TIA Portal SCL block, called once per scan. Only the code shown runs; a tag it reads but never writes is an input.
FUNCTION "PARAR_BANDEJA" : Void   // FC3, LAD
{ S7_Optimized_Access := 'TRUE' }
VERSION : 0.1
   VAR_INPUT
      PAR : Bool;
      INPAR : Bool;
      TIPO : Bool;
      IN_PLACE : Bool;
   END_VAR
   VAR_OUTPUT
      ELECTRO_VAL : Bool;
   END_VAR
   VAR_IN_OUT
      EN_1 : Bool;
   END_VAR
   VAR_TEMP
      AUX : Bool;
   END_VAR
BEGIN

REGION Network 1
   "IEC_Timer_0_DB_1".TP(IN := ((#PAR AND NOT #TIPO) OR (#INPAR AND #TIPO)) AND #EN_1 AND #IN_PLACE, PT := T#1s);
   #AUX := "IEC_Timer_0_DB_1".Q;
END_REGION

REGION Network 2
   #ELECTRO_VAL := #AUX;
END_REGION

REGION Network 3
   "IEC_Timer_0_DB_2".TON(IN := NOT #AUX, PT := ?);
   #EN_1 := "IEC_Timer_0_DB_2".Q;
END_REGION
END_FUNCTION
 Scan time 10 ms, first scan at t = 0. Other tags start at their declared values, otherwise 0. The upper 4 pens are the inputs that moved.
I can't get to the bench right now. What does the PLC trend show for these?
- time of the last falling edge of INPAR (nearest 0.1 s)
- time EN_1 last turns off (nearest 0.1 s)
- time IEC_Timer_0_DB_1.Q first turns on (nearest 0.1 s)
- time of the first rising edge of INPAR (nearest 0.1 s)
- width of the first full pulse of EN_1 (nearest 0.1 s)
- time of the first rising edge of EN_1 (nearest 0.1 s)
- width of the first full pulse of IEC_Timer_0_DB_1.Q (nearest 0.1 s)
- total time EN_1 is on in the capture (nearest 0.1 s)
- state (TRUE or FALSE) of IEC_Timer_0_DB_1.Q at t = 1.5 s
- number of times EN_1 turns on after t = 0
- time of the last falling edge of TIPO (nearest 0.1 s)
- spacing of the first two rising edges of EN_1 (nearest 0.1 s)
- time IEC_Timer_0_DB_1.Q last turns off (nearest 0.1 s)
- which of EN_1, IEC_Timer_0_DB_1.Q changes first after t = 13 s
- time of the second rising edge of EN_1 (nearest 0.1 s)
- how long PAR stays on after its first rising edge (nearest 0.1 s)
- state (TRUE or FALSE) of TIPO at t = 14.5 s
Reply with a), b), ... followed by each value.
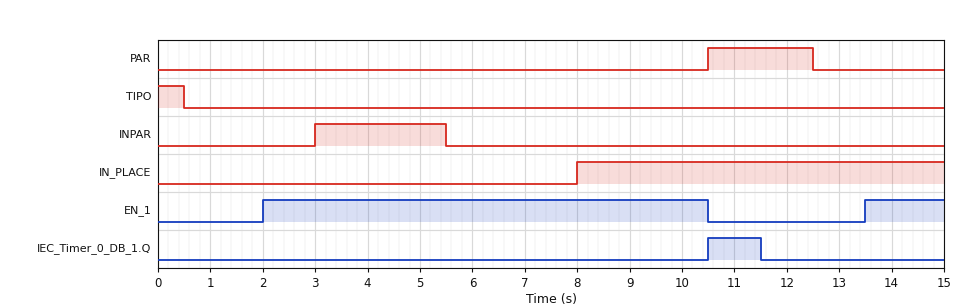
a) 5.5 s
b) 10.5 s
c) 10.5 s
d) 3.0 s
e) 8.5 s
f) 2.0 s
g) 1.0 s
h) 10.0 s
i) FALSE
j) 2
k) 0.5 s
l) 11.5 s
m) 11.5 s
n) EN_1
o) 13.5 s
p) 2.0 s
q) FALSE
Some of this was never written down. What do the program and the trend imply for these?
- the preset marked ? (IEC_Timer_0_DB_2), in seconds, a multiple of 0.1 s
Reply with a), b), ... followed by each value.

a) 2.0 s
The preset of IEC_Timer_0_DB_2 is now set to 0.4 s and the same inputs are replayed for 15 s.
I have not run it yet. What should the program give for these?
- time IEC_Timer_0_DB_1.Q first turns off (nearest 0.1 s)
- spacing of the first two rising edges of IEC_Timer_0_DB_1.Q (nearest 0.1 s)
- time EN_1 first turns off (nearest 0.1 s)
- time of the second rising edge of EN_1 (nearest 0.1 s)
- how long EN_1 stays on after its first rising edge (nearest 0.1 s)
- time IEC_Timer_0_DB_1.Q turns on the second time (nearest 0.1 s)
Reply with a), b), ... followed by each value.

a) 11.5 s
b) 1.4 s
c) 10.5 s
d) 11.9 s
e) 10.1 s
f) 11.9 s
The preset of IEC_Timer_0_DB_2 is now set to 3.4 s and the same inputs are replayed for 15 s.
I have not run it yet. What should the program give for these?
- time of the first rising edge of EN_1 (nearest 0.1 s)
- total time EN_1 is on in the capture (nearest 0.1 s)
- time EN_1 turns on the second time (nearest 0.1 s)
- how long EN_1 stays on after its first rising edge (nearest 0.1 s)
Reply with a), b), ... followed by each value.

a) 3.4 s
b) 7.2 s
c) 14.9 s
d) 7.1 s
